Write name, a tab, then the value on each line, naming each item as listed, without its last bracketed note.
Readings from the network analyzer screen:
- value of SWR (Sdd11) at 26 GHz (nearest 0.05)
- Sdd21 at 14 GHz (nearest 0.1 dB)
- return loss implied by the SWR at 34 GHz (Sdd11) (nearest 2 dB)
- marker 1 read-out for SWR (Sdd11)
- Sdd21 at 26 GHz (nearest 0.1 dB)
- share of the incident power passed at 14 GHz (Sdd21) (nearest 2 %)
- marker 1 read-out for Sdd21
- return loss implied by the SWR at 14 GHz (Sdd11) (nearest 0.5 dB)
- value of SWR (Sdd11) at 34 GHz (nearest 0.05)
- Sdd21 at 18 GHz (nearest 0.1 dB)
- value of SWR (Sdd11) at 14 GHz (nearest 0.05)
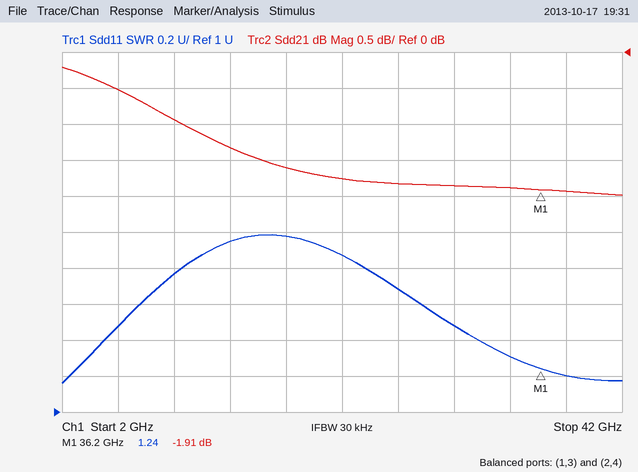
value of SWR (Sdd11) at 26 GHz	1.70
Sdd21 at 14 GHz	-1.3 dB
return loss implied by the SWR at 34 GHz (Sdd11)	18 dB
marker 1 read-out for SWR	1.24
Sdd21 at 26 GHz	-1.8 dB
share of the incident power passed at 14 GHz (Sdd21)	74 %
marker 1 read-out for Sdd21	-1.91 dB
return loss implied by the SWR at 14 GHz (Sdd11)	10.0 dB
value of SWR (Sdd11) at 34 GHz	1.30
Sdd21 at 18 GHz	-1.6 dB
value of SWR (Sdd11) at 14 GHz	1.95
